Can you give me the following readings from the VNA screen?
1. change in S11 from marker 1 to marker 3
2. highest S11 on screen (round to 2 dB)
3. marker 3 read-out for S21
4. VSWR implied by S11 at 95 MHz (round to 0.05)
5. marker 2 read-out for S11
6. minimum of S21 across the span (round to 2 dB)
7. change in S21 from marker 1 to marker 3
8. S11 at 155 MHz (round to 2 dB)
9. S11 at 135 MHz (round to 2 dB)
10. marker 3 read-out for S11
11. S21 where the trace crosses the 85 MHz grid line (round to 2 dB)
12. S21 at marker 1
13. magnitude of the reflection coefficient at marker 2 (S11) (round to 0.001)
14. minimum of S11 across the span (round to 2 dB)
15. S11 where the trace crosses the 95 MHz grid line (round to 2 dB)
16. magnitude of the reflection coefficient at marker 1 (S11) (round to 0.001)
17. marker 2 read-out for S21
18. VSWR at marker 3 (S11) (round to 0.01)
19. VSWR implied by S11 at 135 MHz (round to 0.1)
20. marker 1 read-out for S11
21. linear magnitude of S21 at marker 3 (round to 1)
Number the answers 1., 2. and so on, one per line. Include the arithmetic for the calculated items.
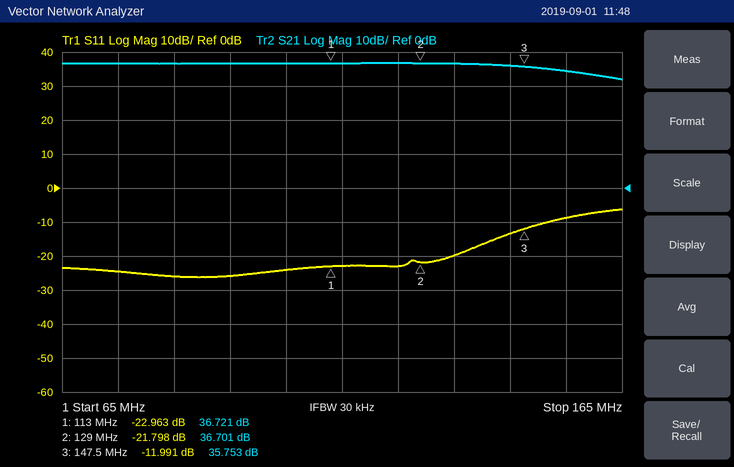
1. -11.991 − (-22.963) = 10.972 dB
2. -6 dB
3. 35.753 dB
4. |Γ| = 10^(-26/20) = 0.0501; VSWR = (1 + 0.0501)/(1 − 0.0501) ≈ 1.11, so 1.10 to the nearest 0.05
5. -21.798 dB
6. 32 dB
7. 35.753 − (36.721) = -0.968 dB
8. -8 dB
9. -20 dB
10. -11.991 dB
11. 36 dB
12. 36.721 dB
13. 10^(-21.798/20) ≈ 0.081
14. -26 dB
15. -26 dB
16. 10^(-22.963/20) ≈ 0.071
17. 36.701 dB
18. (1 + 0.2514)/(1 − 0.2514) ≈ 1.67
19. |Γ| = 10^(-20/20) = 0.1000; VSWR = (1 + 0.1000)/(1 − 0.1000) ≈ 1.2
20. -22.963 dB
21. 10^(35.753/20) ≈ 61
